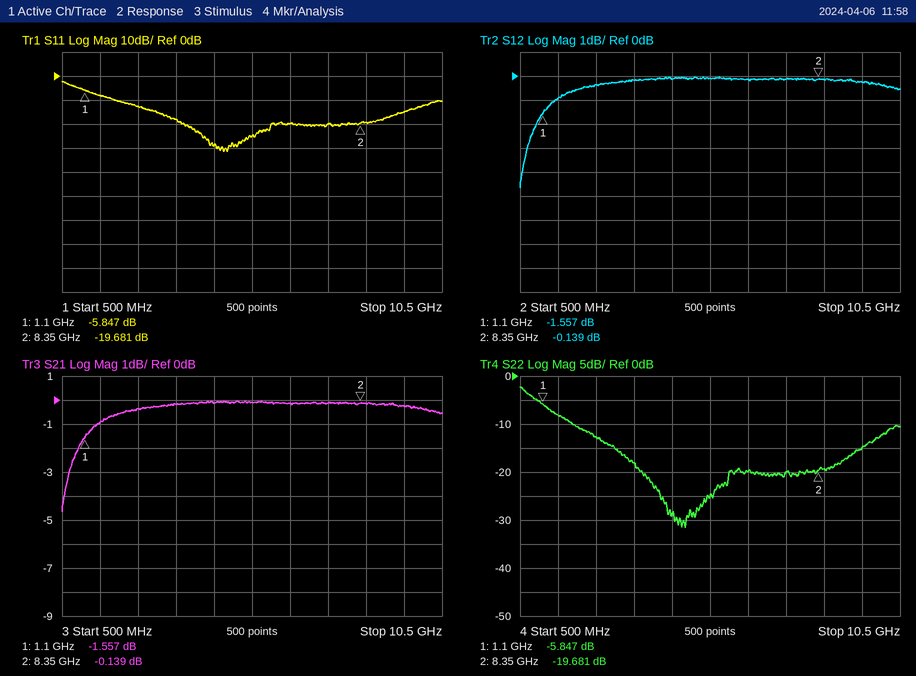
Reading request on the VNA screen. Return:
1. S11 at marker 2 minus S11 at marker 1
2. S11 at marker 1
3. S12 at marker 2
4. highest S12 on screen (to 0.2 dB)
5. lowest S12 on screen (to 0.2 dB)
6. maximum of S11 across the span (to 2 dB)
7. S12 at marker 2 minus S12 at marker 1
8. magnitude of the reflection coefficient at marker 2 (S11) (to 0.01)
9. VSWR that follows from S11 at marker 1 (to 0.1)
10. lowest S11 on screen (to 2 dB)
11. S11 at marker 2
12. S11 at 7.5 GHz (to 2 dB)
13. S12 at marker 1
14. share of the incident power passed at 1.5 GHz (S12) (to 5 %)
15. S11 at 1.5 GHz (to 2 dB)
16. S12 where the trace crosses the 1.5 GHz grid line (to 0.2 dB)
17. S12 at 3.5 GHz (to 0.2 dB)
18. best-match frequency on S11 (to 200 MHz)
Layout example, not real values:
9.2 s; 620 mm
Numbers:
-13.834 dB; -5.847 dB; -0.139 dB; 0.0 dB; -4.6 dB; -2 dB; 1.418 dB; 0.10; 3.1; -32 dB; -19.681 dB; -20 dB; -1.557 dB; 80 %; -8 dB; -1.0 dB; -0.2 dB; 4.8 GHz
